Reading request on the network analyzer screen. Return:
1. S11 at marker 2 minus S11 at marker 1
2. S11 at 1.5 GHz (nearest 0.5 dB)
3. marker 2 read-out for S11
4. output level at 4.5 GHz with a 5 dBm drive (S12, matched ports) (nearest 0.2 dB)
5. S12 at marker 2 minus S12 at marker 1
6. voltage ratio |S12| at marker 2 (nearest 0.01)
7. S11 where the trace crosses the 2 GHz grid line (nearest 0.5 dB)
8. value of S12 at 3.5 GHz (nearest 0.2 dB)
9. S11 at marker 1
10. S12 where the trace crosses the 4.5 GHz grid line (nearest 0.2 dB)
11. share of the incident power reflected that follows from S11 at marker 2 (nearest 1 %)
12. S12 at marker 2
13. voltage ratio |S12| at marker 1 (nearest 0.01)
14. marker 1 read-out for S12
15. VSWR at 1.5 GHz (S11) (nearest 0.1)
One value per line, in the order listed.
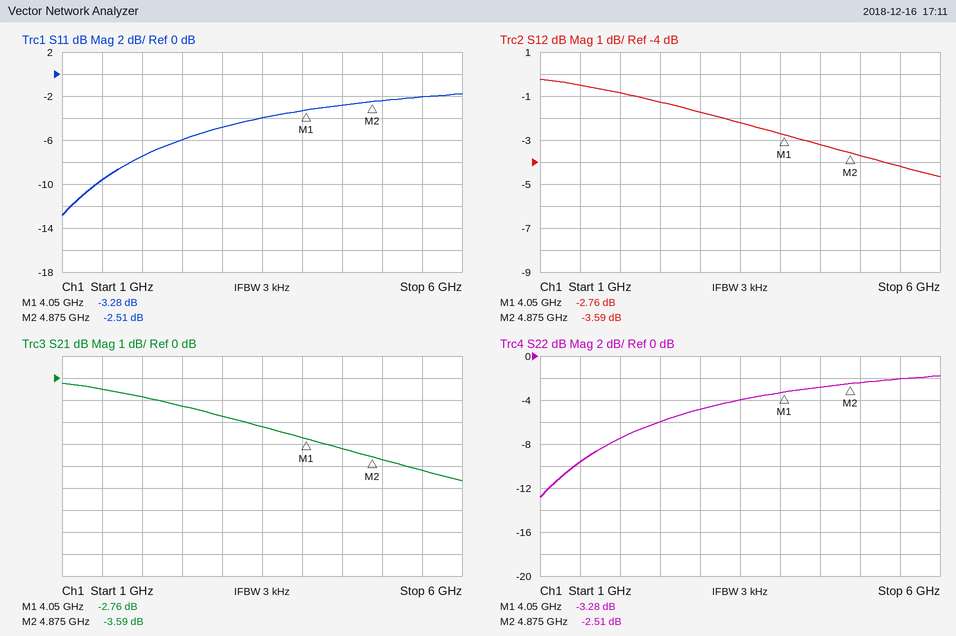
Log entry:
0.77 dB
-9.5 dB
-2.51 dB
1.8 dBm
-0.83 dB
0.66
-7.5 dB
-2.2 dB
-3.28 dB
-3.2 dB
56 %
-3.59 dB
0.73
-2.76 dB
2.0
